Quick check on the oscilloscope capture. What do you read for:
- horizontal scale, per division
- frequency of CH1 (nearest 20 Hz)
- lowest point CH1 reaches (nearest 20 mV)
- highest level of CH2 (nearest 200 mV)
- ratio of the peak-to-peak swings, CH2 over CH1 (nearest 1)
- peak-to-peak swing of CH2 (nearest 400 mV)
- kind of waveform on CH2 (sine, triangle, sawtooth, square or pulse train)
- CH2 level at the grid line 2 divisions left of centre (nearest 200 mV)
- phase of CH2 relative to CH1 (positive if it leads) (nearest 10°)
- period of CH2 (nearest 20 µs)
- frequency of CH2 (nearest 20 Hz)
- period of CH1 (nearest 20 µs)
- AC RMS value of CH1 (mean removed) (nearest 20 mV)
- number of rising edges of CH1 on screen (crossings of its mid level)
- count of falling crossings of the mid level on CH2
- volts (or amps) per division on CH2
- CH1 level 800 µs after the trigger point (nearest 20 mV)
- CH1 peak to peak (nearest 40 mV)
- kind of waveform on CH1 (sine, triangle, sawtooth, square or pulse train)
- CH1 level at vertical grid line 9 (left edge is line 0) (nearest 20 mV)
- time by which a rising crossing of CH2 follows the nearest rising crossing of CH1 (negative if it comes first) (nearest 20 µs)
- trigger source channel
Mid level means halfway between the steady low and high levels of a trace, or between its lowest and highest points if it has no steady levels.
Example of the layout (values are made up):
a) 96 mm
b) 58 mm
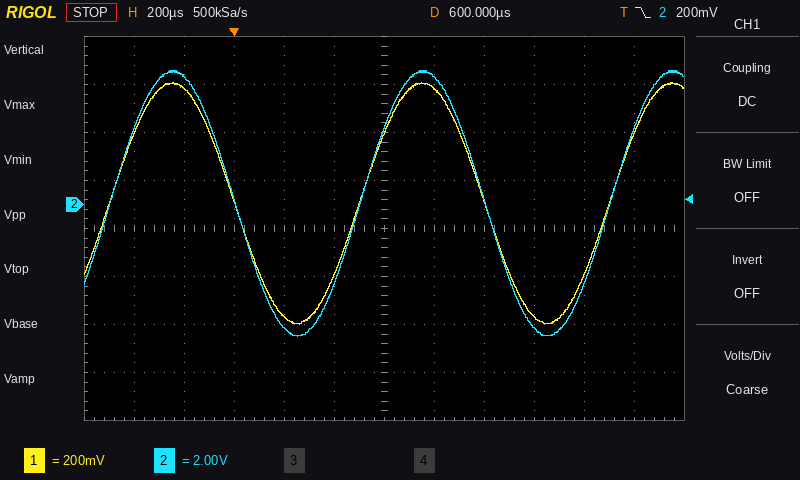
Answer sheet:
a) 200 µs
b) 1.00 kHz
c) -500 mV
d) 5.6 V
e) 11
f) 11.2 V
g) sine
h) -5.2 V
i) 0°
j) 1.00 ms
k) 1.00 kHz
l) 1.00 ms
m) 360 mV
n) 3
o) 2
p) 2 V
q) 480 mV
r) 1.00 V
s) sine
t) -460 mV
u) 0 µs
v) CH2
